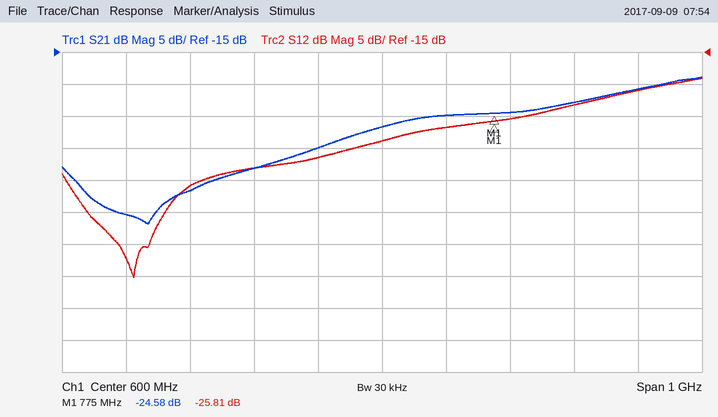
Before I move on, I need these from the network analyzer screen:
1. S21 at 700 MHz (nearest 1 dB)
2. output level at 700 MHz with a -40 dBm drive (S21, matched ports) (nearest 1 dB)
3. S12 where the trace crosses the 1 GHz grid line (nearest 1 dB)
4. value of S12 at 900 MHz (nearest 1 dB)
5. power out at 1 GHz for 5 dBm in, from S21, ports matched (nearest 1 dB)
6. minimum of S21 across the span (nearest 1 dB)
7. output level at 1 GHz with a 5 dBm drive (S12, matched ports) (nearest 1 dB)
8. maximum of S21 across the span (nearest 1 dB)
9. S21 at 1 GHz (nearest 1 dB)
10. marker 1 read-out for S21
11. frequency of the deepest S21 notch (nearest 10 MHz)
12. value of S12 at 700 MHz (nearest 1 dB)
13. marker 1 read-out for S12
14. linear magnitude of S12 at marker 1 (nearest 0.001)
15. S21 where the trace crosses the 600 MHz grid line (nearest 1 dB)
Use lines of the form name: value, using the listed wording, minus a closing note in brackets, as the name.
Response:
S21 at 700 MHz: -25 dB
output level at 700 MHz with a -40 dBm drive (S21, matched ports): -65 dBm
S12 where the trace crosses the 1 GHz grid line: -21 dB
value of S12 at 900 MHz: -23 dB
power out at 1 GHz for 5 dBm in, from S21, ports matched: -16 dBm
minimum of S21 across the span: -42 dB
output level at 1 GHz with a 5 dBm drive (S12, matched ports): -16 dBm
maximum of S21 across the span: -19 dB
S21 at 1 GHz: -21 dB
marker 1 read-out for S21: -24.58 dB
frequency of the deepest S21 notch: 230 MHz
value of S12 at 700 MHz: -27 dB
marker 1 read-out for S12: -25.81 dB
linear magnitude of S12 at marker 1: 0.051
S21 where the trace crosses the 600 MHz grid line: -27 dB
